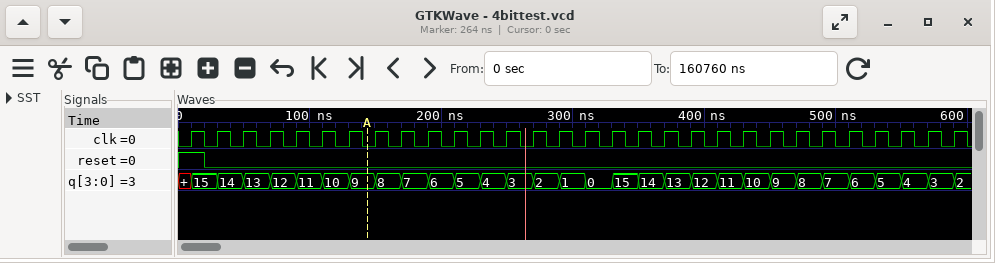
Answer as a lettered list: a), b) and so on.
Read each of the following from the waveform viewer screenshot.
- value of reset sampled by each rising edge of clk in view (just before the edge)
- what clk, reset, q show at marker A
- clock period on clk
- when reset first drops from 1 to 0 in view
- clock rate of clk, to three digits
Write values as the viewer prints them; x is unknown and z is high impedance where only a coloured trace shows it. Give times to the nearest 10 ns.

a) 1 0 0 0 0 0 0 0 0 0 0 0 0 0 0 0 0 0 0 0 0 0 0 0 0 0 0 0 0 0
b) clk=0, reset=0, q=9
c) 20 ns
d) 20 ns
e) 50.0 MHz
